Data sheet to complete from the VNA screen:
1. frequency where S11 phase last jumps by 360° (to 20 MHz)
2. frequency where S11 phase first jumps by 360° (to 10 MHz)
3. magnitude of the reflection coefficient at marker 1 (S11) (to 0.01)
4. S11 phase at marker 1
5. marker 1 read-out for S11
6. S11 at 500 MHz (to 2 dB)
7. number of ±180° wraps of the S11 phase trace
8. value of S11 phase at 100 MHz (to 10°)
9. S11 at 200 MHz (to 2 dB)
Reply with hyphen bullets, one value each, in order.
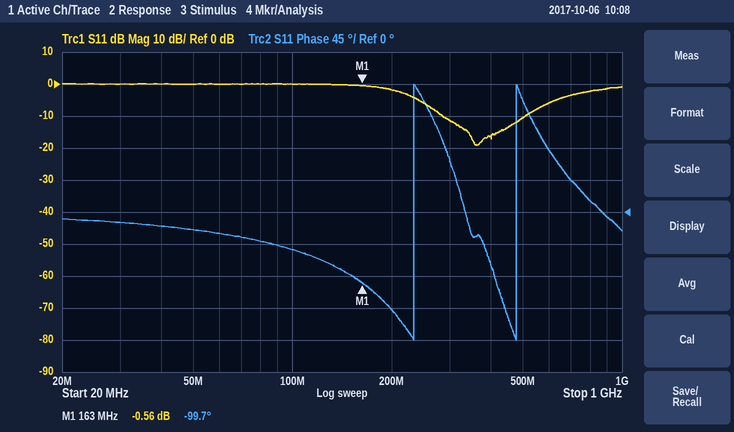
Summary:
- 480 MHz
- 230 MHz
- 0.94
- -99.7°
- -0.56 dB
- -10 dB
- 2
- -50°
- -2 dB
